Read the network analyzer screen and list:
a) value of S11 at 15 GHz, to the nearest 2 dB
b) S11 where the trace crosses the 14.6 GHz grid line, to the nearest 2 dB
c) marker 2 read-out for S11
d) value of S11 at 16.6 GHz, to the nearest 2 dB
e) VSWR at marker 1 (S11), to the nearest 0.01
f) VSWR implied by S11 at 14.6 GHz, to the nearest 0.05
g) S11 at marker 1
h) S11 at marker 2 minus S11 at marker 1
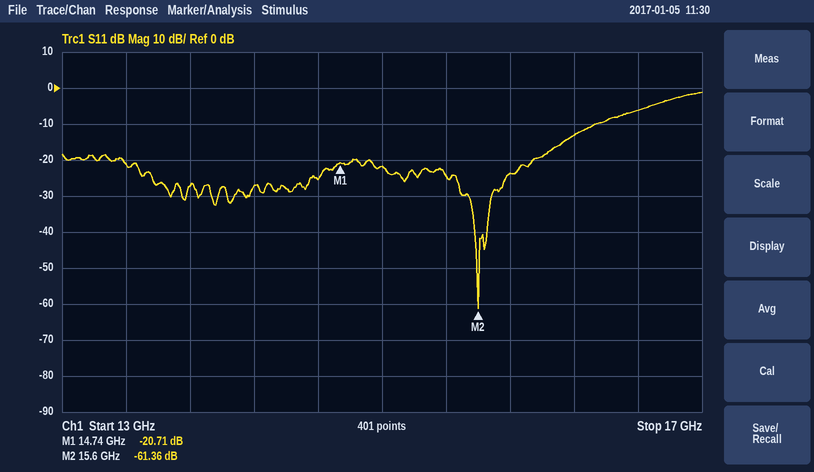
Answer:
-22 dB
-26 dB
-61.36 dB
-6 dB
1.20
1.10
-20.71 dB
-40.65 dB
